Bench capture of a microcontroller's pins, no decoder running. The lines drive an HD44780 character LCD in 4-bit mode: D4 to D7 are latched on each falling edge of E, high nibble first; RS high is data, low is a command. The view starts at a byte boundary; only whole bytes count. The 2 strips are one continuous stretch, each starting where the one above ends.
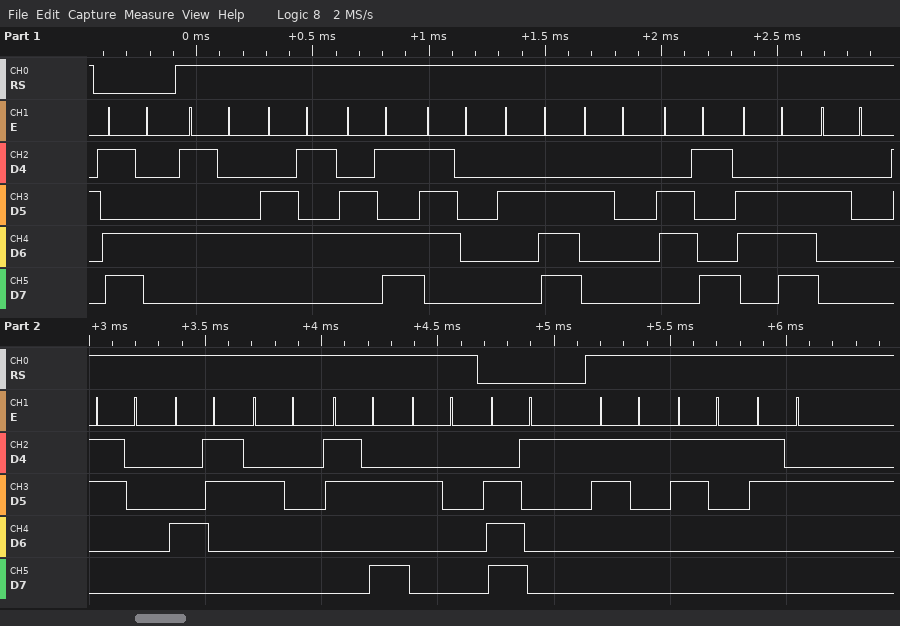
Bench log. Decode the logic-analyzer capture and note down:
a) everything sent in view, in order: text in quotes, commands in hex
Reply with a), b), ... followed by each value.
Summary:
a) 0xD4 "Temp. in 0C : " 0xE1 "112"
